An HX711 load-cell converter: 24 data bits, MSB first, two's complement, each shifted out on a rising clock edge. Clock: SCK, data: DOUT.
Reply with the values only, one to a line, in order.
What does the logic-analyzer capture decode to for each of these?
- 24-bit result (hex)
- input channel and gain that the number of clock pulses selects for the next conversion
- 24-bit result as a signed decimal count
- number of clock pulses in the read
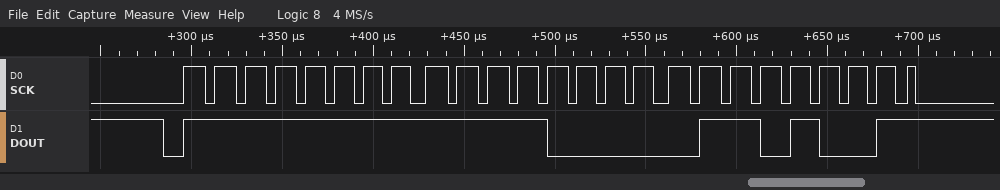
0xFFF069
channel A, gain 128
-3991
25
